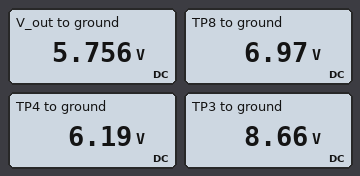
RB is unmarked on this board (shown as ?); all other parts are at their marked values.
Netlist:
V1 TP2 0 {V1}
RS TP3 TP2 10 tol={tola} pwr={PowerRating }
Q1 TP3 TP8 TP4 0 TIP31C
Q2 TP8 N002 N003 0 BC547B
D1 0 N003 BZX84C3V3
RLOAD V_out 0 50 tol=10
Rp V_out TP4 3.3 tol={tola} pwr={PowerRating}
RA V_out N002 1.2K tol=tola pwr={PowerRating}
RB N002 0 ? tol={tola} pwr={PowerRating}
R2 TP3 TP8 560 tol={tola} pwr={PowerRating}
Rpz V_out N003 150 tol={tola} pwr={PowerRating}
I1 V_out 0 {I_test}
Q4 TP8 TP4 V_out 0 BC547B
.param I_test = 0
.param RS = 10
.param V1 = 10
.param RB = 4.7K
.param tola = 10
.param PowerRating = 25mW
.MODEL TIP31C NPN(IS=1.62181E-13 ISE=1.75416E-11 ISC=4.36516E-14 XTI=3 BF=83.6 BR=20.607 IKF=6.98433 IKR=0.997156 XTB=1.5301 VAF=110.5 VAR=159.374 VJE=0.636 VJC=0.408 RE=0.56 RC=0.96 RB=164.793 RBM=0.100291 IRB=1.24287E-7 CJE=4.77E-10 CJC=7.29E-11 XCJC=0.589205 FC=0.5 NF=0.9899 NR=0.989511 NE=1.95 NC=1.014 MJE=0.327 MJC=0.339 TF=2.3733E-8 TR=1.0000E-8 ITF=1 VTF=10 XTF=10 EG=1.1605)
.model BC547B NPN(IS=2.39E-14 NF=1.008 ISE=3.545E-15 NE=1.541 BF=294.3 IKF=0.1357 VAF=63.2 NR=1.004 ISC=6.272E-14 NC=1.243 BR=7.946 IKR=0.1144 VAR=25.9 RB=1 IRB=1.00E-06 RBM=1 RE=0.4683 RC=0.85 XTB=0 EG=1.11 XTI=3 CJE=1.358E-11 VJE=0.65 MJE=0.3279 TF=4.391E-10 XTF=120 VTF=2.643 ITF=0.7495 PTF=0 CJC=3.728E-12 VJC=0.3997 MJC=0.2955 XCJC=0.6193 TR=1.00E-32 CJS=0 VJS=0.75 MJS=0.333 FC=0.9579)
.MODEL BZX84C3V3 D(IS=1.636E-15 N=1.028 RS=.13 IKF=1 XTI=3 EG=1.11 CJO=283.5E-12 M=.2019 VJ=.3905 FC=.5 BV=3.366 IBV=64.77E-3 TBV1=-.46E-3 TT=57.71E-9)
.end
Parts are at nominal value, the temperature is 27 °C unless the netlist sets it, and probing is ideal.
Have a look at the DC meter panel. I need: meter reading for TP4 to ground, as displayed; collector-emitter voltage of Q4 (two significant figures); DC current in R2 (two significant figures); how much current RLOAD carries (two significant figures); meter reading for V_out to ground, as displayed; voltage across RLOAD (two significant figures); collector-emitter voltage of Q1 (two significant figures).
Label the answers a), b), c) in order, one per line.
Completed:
a) 6.19 V
b) 1.2 V
c) 3.0 mA
d) 120 mA
e) 5.756 V
f) 5.8 V
g) 2.5 V
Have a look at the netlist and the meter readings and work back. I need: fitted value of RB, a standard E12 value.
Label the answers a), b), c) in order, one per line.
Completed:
a) 2.7 kΩ
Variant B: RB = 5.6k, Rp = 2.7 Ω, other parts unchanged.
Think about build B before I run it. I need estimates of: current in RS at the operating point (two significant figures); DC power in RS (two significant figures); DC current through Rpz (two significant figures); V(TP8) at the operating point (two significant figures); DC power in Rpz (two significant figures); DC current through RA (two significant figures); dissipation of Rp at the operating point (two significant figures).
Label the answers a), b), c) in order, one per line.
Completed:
a) 110 mA
b) 130 mW
c) 10 mA
d) 5.9 V
e) 16 mW
f) 730 µA
g) 32 mW
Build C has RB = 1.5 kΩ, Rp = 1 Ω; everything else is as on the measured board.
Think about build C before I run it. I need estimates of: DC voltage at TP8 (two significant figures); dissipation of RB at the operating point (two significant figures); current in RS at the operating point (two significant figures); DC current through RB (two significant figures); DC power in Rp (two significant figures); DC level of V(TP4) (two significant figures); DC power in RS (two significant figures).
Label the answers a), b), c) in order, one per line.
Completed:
a) 7.4 V
b) 8.6 mW
c) 150 mA
d) 2.4 mA
e) 23 mW
f) 6.6 V
g) 230 mW
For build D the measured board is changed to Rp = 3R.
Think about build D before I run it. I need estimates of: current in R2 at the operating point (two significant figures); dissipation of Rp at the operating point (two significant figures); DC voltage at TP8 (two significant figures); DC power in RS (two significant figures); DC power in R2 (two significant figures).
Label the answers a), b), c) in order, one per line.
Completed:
a) 3.1 mA
b) 53 mW
c) 6.9 V
d) 180 mW
e) 5.3 mW
